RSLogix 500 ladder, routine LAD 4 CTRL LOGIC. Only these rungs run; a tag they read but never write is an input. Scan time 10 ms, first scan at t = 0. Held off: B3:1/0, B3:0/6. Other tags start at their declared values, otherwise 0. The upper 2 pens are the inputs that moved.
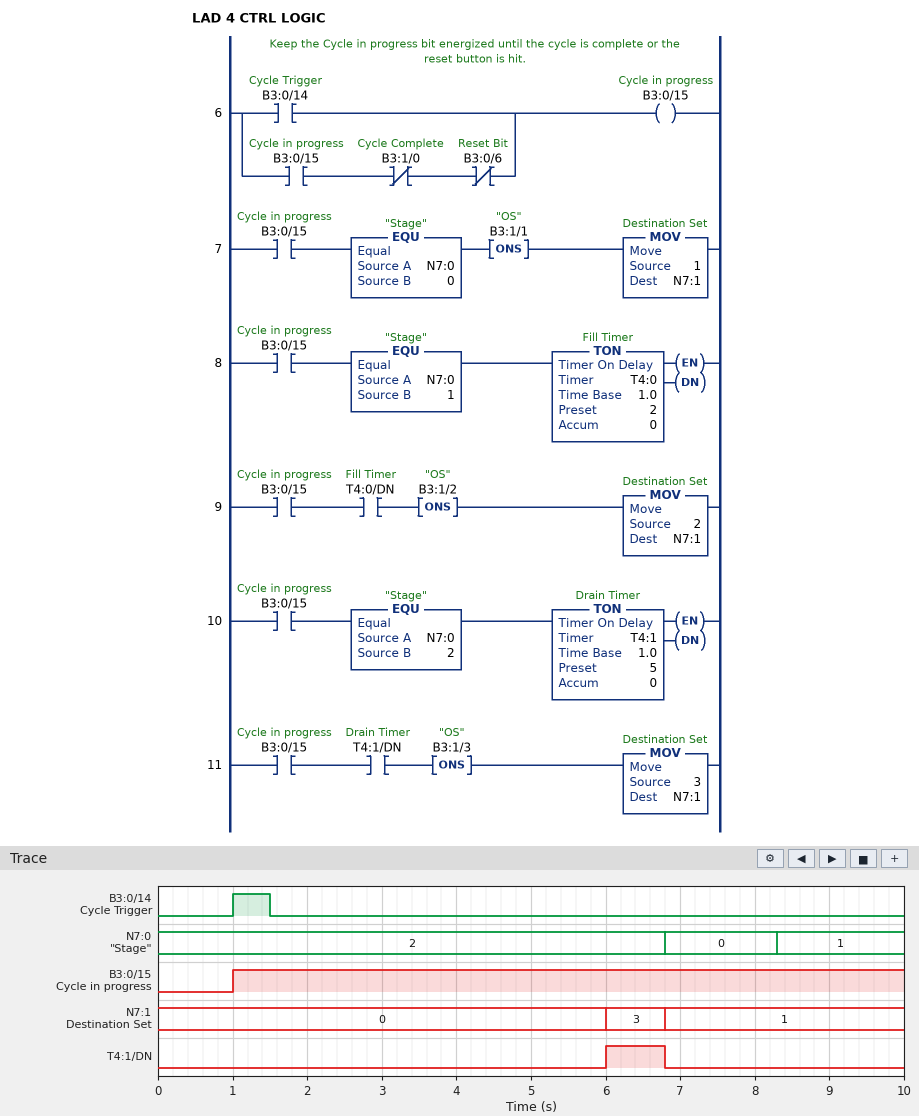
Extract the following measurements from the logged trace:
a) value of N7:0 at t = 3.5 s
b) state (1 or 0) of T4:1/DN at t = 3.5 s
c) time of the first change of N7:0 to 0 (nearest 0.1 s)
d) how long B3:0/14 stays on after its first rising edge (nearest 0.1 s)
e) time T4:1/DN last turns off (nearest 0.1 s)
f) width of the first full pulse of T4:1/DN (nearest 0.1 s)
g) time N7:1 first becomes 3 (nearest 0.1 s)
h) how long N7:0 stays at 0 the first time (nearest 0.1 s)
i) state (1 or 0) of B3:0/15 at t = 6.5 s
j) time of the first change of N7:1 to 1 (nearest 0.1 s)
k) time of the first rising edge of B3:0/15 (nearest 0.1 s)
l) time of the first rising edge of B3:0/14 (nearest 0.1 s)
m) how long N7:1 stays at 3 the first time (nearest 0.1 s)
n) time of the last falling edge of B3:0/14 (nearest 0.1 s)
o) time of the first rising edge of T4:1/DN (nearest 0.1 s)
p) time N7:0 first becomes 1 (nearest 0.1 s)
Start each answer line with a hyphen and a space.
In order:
- 2
- 0
- 6.8 s
- 0.5 s
- 6.8 s
- 0.8 s
- 6.0 s
- 1.5 s
- 1
- 6.8 s
- 1.0 s
- 1.0 s
- 0.8 s
- 1.5 s
- 6.0 s
- 8.3 s
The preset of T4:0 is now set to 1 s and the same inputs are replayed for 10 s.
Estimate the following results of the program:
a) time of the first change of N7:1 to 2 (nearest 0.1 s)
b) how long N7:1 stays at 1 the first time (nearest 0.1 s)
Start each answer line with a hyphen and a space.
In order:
- 9.3 s
- 2.5 s
